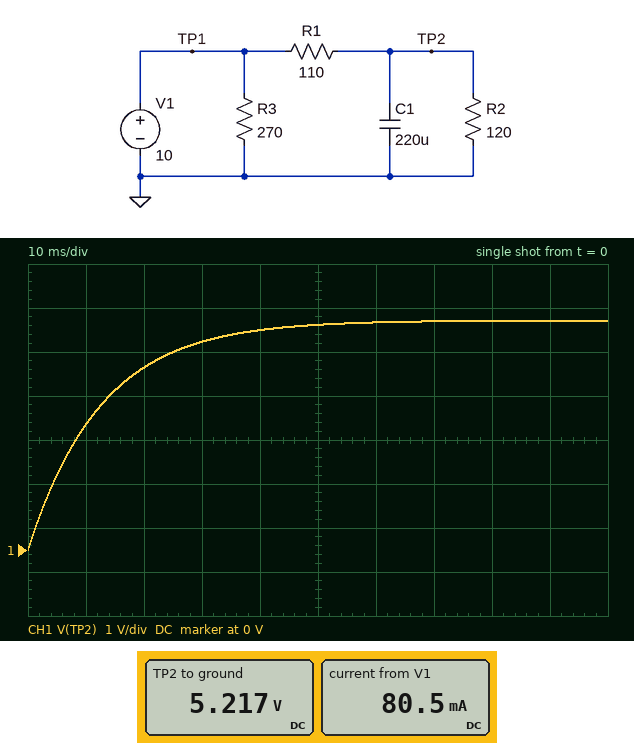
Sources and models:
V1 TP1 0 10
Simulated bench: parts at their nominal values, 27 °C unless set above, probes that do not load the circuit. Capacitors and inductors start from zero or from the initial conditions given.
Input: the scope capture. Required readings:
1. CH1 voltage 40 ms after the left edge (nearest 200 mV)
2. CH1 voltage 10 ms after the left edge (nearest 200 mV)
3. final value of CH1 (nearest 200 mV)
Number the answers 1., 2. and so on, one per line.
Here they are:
1. 5.0 V
2. 2.8 V
3. 5.2 V
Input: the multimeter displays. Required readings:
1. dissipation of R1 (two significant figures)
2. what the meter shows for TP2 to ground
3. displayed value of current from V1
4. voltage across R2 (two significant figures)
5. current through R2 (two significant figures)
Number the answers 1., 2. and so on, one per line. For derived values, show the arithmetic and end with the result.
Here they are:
1. (10 V - 5.217 V)^2 / 110 Ω = 210 mW
2. 5.217 V
3. 80.5 mA
4. 5.217 V = 5.2 V
5. (5.217 V) / 120 Ω = 43 mA
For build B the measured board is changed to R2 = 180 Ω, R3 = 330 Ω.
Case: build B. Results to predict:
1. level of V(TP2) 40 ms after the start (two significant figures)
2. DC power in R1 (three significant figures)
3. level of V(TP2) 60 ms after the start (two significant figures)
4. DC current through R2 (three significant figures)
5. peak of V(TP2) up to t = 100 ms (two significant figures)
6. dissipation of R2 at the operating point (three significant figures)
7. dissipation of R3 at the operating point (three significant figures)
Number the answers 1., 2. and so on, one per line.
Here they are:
1. 5.8 V
2. 131 mW
3. 6.1 V
4. 34.5 mA
5. 6.2 V
6. 214 mW
7. 303 mW
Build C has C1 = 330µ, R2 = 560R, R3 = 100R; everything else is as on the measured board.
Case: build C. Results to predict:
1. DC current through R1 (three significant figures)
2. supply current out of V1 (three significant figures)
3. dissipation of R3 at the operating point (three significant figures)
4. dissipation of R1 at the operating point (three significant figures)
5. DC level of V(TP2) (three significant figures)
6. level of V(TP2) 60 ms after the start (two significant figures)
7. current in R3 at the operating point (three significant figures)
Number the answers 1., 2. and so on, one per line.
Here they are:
1. 14.9 mA
2. 115 mA
3. 1.00 W
4. 24.5 mW
5. 8.36 V
6. 7.2 V
7. 100 mA
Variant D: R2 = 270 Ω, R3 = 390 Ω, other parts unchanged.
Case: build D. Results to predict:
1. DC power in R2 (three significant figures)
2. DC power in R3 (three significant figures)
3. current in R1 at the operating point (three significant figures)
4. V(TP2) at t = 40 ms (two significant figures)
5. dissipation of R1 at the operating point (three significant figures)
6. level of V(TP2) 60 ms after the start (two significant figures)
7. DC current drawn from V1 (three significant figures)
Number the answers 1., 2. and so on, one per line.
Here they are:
1. 187 mW
2. 256 mW
3. 26.3 mA
4. 6.4 V
5. 76.2 mW
6. 6.9 V
7. 52.0 mA
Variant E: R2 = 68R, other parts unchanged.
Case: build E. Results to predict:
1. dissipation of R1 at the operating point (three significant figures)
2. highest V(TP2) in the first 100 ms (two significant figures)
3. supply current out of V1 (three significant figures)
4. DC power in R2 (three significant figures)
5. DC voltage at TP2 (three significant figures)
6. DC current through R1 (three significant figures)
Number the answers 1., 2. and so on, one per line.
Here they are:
1. 347 mW
2. 3.8 V
3. 93.2 mA
4. 215 mW
5. 3.82 V
6. 56.2 mA
